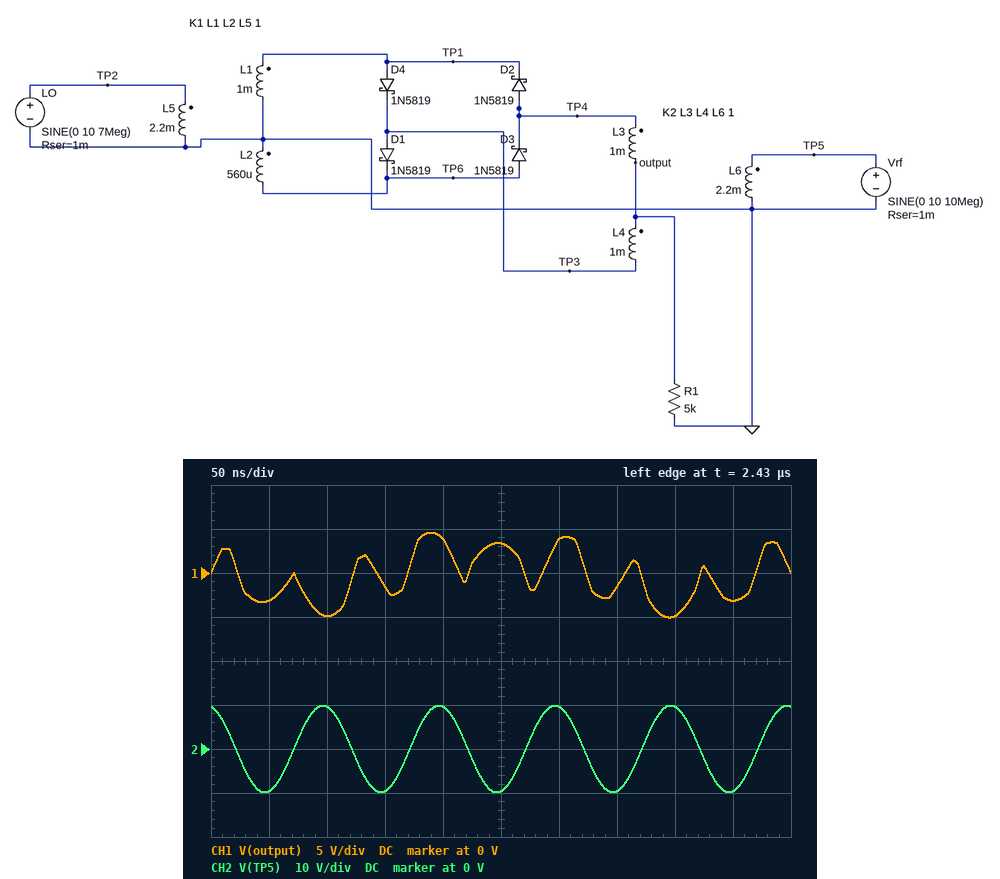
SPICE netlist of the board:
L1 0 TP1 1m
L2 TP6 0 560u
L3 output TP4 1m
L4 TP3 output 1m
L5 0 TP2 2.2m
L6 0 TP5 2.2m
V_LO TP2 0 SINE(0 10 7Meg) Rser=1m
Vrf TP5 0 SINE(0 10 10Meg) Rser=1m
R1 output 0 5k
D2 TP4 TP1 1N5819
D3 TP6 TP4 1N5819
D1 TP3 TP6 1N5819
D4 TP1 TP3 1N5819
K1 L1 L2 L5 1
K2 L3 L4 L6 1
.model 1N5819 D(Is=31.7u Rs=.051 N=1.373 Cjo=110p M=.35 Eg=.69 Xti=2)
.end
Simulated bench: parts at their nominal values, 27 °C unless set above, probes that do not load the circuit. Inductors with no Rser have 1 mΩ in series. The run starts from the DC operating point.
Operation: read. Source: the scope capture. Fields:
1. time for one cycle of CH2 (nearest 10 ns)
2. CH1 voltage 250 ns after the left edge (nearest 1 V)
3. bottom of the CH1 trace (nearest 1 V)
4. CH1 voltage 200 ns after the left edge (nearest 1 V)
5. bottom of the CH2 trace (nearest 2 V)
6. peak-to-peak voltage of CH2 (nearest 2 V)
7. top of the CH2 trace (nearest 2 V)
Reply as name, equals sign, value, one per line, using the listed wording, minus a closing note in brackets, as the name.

time for one cycle of CH2 = 100 ns
CH1 voltage 250 ns after the left edge = 3 V
bottom of the CH1 trace = -5 V
CH1 voltage 200 ns after the left edge = 4 V
bottom of the CH2 trace = -10 V
peak-to-peak voltage of CH2 = 20 V
top of the CH2 trace = 10 V
